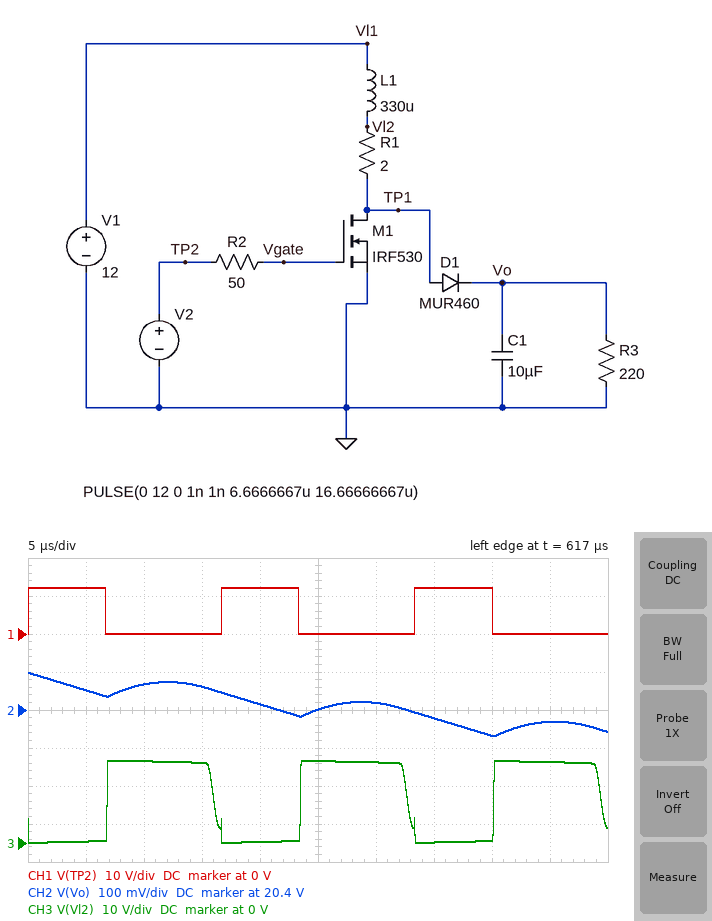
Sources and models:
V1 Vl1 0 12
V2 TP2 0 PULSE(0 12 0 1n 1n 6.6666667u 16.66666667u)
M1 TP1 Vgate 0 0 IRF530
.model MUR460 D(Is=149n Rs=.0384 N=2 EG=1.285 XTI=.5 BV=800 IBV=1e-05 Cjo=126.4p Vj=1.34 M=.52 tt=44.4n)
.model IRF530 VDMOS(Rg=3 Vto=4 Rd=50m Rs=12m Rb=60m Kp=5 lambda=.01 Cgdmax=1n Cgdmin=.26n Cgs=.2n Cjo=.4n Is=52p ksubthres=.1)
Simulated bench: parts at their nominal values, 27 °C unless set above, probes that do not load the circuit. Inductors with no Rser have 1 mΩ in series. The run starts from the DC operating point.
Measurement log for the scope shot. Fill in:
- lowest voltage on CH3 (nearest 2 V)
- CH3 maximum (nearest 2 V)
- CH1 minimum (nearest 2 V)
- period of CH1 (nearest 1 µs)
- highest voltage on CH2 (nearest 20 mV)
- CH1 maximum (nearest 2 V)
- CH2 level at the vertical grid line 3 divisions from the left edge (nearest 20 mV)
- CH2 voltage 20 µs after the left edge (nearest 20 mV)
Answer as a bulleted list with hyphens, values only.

- 0 V
- 22 V
- 0 V
- 17 µs
- 20.50 V
- 12 V
- 20.46 V
- 20.42 V
